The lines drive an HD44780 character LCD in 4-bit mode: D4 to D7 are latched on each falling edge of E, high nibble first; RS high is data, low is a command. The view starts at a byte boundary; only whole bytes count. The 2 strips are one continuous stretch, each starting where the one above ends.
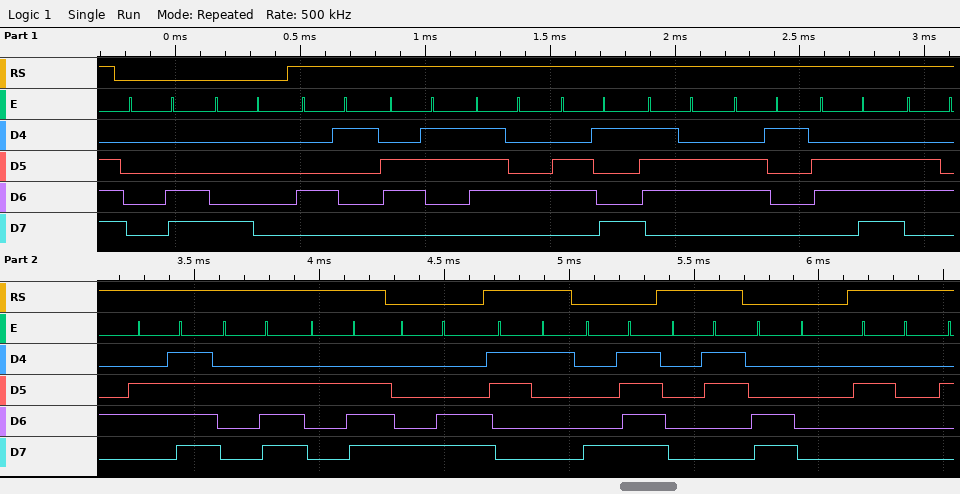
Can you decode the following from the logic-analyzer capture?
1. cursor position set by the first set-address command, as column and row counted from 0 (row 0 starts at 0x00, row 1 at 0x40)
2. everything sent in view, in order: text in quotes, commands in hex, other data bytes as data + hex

column 0, row 0
0x0C 0x80 "Activando.." 0x8C "1" 0x8F data 03 0xC0 " "
